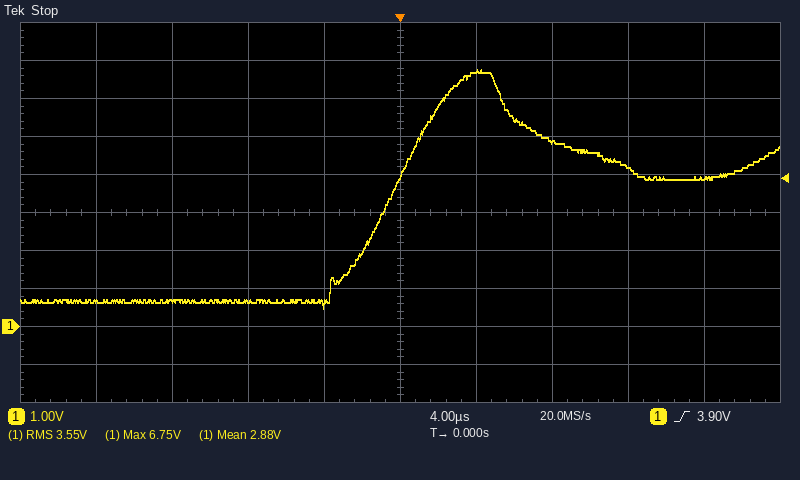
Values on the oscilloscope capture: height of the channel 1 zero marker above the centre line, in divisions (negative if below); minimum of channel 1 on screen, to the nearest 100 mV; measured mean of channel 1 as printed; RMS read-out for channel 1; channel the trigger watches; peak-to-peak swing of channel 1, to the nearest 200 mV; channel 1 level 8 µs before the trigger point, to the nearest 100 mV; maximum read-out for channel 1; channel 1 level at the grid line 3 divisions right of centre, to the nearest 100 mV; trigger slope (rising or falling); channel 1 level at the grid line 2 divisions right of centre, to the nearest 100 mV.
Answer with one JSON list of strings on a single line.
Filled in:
["-3.0 div", "500 mV", "2.88 V", "3.55 V", "channel 1", "6.2 V", "700 mV", "6.75 V", "4.2 V", "rising", "4.9 V"]
